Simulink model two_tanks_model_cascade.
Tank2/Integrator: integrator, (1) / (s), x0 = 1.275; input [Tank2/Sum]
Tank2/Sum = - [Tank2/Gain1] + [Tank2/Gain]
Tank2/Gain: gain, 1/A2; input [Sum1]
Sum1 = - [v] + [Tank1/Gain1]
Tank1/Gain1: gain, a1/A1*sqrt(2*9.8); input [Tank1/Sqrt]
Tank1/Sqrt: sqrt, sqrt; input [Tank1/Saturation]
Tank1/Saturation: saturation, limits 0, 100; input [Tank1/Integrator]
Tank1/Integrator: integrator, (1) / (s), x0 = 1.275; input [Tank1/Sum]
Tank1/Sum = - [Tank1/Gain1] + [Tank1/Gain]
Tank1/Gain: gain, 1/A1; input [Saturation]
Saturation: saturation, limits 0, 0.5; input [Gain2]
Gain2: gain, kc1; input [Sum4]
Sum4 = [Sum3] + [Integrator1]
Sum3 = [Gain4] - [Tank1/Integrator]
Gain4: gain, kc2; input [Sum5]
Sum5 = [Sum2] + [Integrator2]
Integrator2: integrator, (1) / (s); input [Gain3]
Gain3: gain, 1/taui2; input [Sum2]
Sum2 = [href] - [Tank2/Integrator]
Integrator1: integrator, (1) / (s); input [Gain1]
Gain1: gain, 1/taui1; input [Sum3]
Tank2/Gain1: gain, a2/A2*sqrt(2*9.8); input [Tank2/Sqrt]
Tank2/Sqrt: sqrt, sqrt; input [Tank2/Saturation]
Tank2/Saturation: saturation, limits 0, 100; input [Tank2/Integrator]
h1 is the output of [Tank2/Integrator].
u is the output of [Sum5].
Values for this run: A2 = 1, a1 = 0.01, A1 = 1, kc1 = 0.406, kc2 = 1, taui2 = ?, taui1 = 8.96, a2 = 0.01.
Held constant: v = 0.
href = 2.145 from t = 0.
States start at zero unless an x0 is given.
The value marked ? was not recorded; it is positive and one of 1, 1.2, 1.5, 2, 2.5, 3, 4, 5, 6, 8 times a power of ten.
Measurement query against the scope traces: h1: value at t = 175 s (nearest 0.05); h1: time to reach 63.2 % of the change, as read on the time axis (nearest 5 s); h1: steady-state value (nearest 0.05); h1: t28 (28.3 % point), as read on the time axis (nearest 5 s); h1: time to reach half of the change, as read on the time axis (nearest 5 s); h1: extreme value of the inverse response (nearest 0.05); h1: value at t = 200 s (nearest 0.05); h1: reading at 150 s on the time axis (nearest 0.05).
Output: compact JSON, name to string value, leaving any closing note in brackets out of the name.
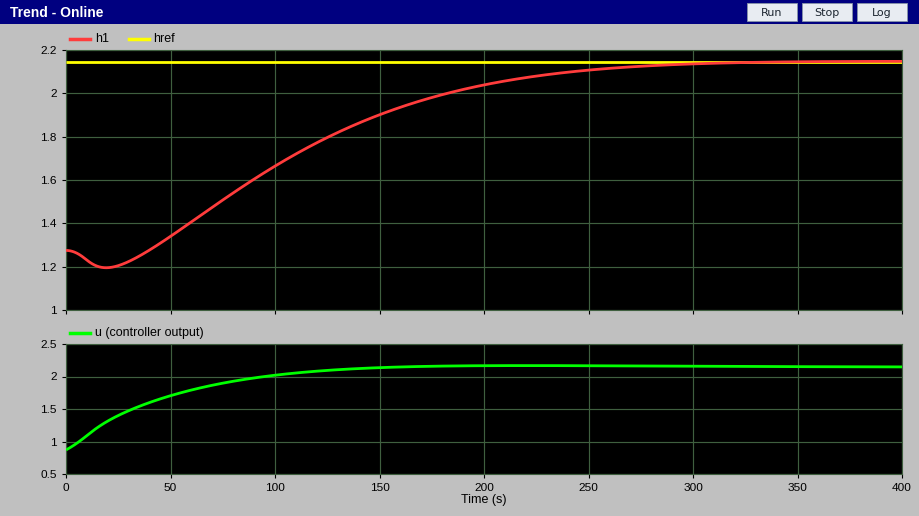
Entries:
{"h1: value at t = 175 s": "2.00", "h1: time to reach 63.2 % of the change, as read on the time axis": "130 s", "h1: steady-state value": "2.15", "h1: t28 (28.3 % point), as read on the time axis": "75 s", "h1: time to reach half of the change, as read on the time axis": "110 s", "h1: extreme value of the inverse response": "1.20", "h1: value at t = 200 s": "2.05", "h1: reading at 150 s on the time axis": "1.90"}
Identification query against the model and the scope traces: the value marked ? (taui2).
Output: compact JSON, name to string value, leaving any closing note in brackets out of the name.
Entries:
{"the value marked ?": "50"}
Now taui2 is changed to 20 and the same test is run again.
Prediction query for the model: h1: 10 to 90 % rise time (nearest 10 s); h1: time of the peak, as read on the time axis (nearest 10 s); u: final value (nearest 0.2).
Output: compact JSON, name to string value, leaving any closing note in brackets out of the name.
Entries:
{"h1: 10 to 90 % rise time": "60 s", "h1: time of the peak, as read on the time axis": "150 s", "u: final value": "2.2"}
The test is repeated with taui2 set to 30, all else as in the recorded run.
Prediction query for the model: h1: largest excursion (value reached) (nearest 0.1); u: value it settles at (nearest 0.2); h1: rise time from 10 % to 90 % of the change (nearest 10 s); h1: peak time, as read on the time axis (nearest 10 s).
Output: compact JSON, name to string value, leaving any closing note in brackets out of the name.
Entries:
{"h1: largest excursion (value reached)": "2.2", "u: value it settles at": "2.2", "h1: rise time from 10 % to 90 % of the change": "90 s", "h1: peak time, as read on the time axis": "200 s"}
